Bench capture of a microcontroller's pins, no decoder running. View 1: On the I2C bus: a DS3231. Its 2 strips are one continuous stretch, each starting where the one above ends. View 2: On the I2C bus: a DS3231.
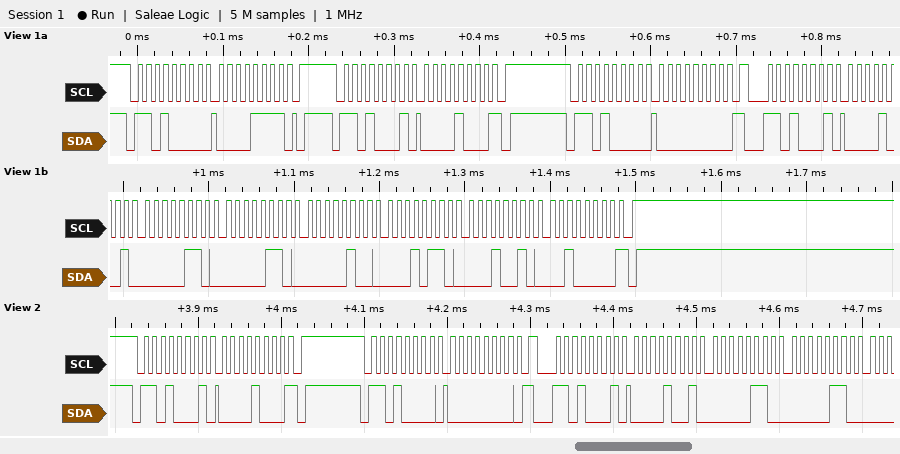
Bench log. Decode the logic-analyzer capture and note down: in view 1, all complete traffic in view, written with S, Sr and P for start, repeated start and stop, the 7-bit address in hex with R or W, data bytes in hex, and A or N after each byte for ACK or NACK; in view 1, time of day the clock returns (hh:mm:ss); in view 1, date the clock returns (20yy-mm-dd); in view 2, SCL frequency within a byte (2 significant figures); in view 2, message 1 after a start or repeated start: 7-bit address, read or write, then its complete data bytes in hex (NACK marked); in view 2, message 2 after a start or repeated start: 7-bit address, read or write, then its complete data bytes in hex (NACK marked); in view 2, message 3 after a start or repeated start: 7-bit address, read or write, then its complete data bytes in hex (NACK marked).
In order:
S 68W A 0F A P S 68R A 08 N P S 68W A 00 A Sr 68R A 09 A 06 A 06 A 04 A 16 A 12 A 20 N P
06:06:09
2020-12-16
100 kHz
0x68 read: 08 NACK
0x68 write: 00
0x68 read: 09 06 06
